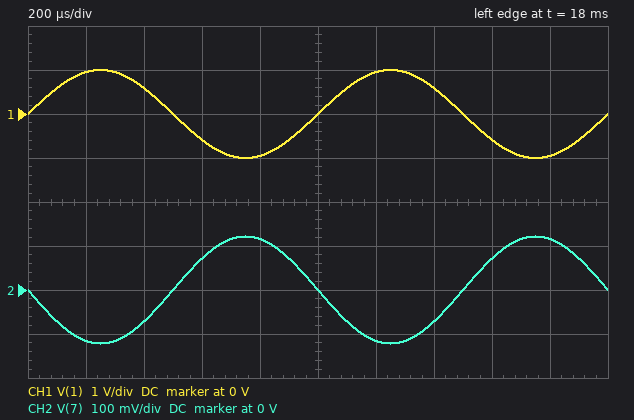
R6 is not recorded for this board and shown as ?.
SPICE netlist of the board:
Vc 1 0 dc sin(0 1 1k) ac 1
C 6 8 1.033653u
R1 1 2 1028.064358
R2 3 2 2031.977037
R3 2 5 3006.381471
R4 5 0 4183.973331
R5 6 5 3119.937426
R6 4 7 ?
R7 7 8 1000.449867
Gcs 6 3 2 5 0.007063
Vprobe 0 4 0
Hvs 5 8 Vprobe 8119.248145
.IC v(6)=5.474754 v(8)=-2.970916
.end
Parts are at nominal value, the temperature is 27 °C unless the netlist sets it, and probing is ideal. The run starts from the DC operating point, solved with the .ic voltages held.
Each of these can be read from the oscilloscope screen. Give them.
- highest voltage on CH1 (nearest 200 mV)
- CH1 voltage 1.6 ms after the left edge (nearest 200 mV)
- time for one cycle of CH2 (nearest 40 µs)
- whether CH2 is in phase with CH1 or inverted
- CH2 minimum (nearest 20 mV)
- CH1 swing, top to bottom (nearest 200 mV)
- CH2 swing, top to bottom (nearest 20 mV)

1.0 V
-600 mV
1.00 ms
inverted
-120 mV
2.0 V
240 mV
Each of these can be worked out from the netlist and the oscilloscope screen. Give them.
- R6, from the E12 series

820 Ω
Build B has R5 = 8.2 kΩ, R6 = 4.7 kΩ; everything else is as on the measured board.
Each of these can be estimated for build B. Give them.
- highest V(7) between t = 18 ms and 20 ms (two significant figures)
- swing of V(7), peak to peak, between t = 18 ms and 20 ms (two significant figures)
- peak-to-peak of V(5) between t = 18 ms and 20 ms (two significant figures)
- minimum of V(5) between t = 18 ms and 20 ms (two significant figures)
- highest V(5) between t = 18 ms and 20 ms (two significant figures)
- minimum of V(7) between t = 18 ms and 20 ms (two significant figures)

2.3 V
4.6 V
2.4 V
-1.2 V
1.2 V
-2.3 V
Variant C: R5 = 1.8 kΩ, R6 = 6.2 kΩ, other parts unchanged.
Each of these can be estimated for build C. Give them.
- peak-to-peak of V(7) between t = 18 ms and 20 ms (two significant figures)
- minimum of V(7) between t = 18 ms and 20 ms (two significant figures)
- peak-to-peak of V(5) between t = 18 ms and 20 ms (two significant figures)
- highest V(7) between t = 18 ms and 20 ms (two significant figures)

53 V
-27 V
7.9 V
27 V
